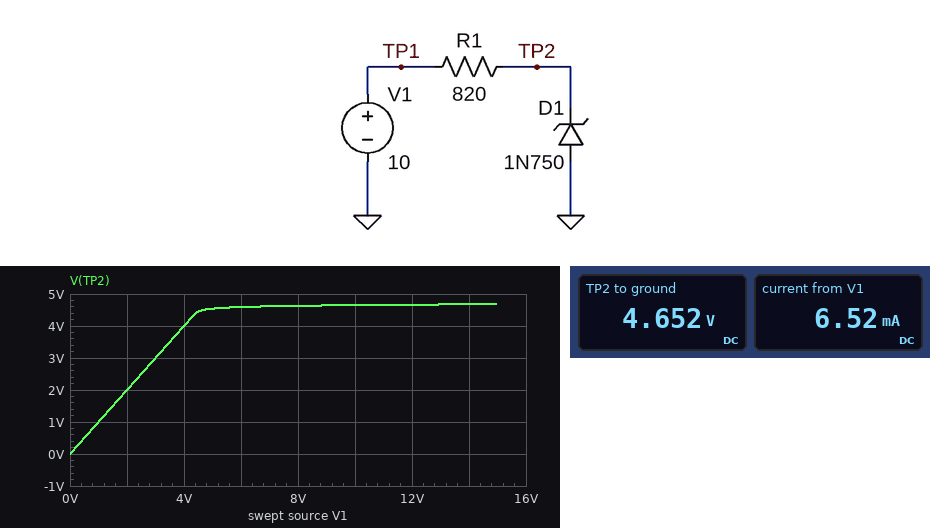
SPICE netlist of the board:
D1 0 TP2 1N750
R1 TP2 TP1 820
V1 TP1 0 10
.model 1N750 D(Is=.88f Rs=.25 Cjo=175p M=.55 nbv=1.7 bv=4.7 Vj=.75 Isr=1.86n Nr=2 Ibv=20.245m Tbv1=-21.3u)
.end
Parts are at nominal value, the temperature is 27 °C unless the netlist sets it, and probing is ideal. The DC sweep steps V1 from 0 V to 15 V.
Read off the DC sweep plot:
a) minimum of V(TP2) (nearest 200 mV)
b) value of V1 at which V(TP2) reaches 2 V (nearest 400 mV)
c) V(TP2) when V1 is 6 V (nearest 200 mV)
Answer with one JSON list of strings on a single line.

["0 V", "2.0 V", "4.6 V"]
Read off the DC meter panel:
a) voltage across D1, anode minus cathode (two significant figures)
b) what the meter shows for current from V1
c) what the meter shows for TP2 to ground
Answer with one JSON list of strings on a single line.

["-4.7 V", "6.52 mA", "4.652 V"]
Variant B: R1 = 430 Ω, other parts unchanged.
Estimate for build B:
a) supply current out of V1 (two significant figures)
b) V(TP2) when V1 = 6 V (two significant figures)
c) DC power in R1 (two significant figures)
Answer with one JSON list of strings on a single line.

["12 mA", "4.6 V", "66 mW"]
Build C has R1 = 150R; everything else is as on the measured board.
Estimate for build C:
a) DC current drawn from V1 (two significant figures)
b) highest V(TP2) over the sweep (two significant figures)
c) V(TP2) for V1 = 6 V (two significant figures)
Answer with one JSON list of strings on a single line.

["35 mA", "4.8 V", "4.7 V"]
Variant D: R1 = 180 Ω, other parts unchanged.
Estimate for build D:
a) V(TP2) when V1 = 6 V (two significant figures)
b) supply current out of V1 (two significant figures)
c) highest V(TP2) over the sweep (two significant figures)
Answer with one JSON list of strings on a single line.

["4.7 V", "29 mA", "4.8 V"]
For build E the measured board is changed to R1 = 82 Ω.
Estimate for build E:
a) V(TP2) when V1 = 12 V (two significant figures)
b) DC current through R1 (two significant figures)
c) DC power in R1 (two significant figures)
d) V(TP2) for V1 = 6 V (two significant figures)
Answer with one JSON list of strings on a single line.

["4.8 V", "64 mA", "330 mW", "4.7 V"]
